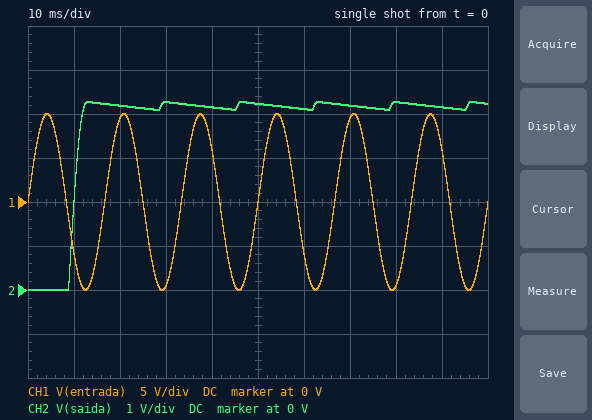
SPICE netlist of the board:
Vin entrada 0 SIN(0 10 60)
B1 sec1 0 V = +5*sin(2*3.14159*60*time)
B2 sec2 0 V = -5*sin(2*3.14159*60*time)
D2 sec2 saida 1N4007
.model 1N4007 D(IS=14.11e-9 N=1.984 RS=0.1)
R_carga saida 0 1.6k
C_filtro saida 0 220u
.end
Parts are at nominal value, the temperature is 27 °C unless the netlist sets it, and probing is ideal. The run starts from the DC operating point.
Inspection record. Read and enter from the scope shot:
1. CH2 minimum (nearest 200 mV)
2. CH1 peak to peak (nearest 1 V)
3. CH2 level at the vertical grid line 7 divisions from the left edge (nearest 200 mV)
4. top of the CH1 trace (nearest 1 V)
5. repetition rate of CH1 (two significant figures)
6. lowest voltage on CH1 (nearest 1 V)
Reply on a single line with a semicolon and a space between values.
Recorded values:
0 V; 20 V; 4.2 V; 10 V; 60 Hz; -10 V
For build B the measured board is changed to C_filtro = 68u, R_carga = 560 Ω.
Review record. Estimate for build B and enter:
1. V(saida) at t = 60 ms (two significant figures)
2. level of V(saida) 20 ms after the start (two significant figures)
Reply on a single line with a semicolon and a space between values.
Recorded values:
3.0 V; 3.6 V
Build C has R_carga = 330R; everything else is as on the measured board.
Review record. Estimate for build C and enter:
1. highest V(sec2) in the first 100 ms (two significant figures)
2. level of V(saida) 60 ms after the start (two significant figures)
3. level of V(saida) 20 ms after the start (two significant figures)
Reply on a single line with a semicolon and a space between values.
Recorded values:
5.0 V; 3.5 V; 3.9 V
